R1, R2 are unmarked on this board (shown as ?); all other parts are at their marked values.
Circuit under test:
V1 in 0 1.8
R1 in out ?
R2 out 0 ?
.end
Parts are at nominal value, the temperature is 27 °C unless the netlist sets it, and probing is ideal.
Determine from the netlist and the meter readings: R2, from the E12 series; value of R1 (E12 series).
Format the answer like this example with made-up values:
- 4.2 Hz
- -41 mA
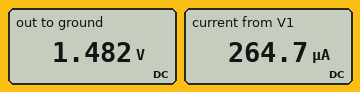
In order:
- 5.6 kΩ
- 1.2 kΩ
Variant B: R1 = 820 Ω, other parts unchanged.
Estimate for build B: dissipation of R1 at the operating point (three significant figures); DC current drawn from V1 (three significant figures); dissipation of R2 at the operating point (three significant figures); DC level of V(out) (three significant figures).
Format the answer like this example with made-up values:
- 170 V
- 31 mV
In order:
- 64.5 µW
- 280 µA
- 440 µW
- 1.57 V
